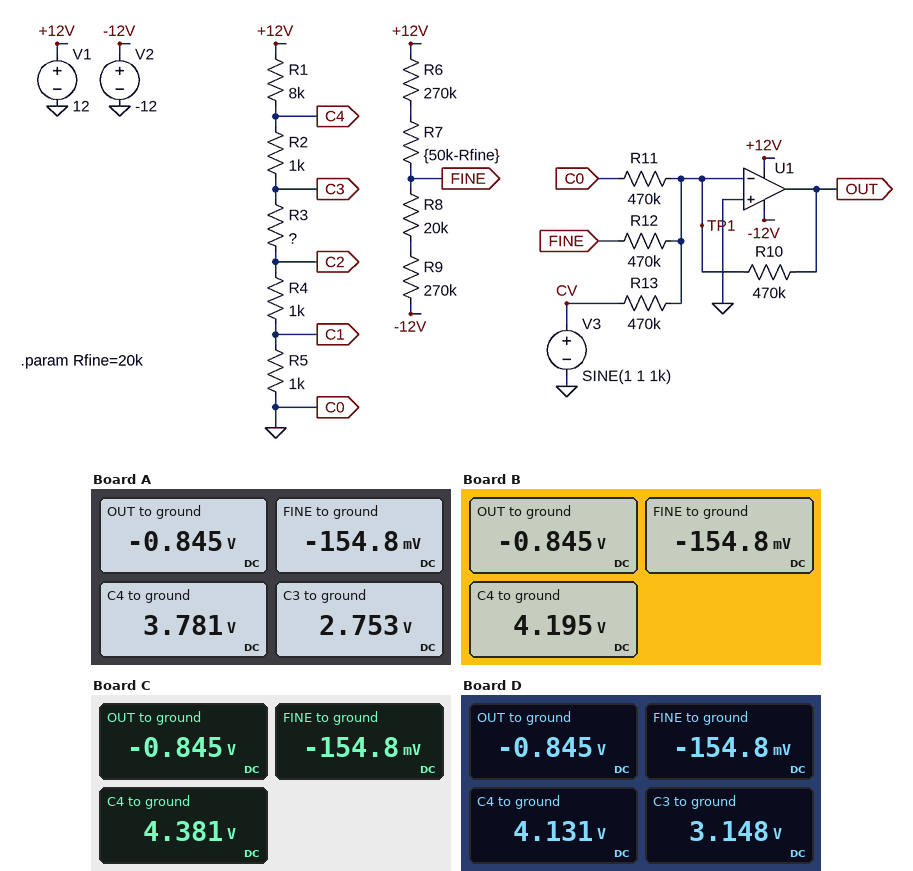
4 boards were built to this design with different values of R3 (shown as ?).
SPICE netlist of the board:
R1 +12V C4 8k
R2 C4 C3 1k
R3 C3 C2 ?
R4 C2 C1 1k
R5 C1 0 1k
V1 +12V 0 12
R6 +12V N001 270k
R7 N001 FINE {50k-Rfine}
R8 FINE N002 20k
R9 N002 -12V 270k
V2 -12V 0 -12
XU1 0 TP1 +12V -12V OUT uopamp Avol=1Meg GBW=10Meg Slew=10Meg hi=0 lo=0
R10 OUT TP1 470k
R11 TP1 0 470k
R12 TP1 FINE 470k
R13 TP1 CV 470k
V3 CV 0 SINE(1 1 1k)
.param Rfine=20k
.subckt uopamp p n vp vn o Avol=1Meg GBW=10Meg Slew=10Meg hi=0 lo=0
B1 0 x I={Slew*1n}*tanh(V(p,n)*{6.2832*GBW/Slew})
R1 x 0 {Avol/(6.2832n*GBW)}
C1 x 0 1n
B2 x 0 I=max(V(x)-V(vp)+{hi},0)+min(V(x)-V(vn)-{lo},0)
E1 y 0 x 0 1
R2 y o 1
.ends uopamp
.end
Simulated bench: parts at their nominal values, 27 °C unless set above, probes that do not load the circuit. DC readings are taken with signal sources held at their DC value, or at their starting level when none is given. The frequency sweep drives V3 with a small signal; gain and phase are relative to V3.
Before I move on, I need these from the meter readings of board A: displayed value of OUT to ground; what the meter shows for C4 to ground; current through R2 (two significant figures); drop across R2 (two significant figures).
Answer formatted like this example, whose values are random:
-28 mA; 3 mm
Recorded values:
-0.845 V; 3.781 V; 1.0 mA; 1.0 V
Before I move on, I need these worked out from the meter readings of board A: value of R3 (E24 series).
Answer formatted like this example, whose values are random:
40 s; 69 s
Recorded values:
680 Ω
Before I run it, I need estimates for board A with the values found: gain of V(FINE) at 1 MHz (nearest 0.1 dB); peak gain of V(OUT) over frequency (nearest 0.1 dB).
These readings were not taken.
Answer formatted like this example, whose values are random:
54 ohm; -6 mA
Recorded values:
-33.0 dB; 0 dB
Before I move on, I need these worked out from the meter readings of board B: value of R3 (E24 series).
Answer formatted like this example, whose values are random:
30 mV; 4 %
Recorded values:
1.3 kΩ
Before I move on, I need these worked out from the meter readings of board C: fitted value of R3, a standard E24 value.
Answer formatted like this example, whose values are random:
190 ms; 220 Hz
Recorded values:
1.6 kΩ
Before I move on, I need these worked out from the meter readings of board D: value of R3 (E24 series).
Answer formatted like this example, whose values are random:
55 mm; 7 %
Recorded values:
1.2 kΩ
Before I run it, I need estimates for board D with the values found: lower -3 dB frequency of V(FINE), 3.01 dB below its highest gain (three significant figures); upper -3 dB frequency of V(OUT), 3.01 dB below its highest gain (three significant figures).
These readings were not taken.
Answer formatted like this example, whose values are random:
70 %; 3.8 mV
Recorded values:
2.66 MHz; 2.66 MHz
